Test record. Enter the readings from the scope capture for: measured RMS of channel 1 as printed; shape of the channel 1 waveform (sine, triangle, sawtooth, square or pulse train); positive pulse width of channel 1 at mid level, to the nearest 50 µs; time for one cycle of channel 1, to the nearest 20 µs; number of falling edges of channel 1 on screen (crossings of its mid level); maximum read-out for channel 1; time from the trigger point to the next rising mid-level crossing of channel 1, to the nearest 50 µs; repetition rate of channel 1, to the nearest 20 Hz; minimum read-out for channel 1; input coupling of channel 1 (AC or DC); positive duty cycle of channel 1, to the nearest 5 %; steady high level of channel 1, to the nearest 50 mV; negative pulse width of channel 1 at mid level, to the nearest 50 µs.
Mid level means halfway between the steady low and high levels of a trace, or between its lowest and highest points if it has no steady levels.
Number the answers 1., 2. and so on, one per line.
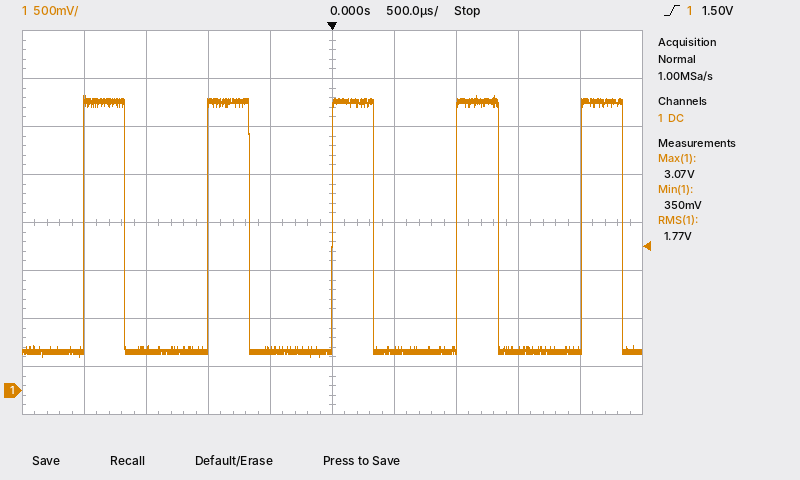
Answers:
1. 1.77 V
2. pulse train
3. 350 µs
4. 1.00 ms
5. 5
6. 3.07 V
7. 1.00 ms
8. 1.00 kHz
9. 350 mV
10. DC
11. 35 %
12. 3.00 V
13. 650 µs
